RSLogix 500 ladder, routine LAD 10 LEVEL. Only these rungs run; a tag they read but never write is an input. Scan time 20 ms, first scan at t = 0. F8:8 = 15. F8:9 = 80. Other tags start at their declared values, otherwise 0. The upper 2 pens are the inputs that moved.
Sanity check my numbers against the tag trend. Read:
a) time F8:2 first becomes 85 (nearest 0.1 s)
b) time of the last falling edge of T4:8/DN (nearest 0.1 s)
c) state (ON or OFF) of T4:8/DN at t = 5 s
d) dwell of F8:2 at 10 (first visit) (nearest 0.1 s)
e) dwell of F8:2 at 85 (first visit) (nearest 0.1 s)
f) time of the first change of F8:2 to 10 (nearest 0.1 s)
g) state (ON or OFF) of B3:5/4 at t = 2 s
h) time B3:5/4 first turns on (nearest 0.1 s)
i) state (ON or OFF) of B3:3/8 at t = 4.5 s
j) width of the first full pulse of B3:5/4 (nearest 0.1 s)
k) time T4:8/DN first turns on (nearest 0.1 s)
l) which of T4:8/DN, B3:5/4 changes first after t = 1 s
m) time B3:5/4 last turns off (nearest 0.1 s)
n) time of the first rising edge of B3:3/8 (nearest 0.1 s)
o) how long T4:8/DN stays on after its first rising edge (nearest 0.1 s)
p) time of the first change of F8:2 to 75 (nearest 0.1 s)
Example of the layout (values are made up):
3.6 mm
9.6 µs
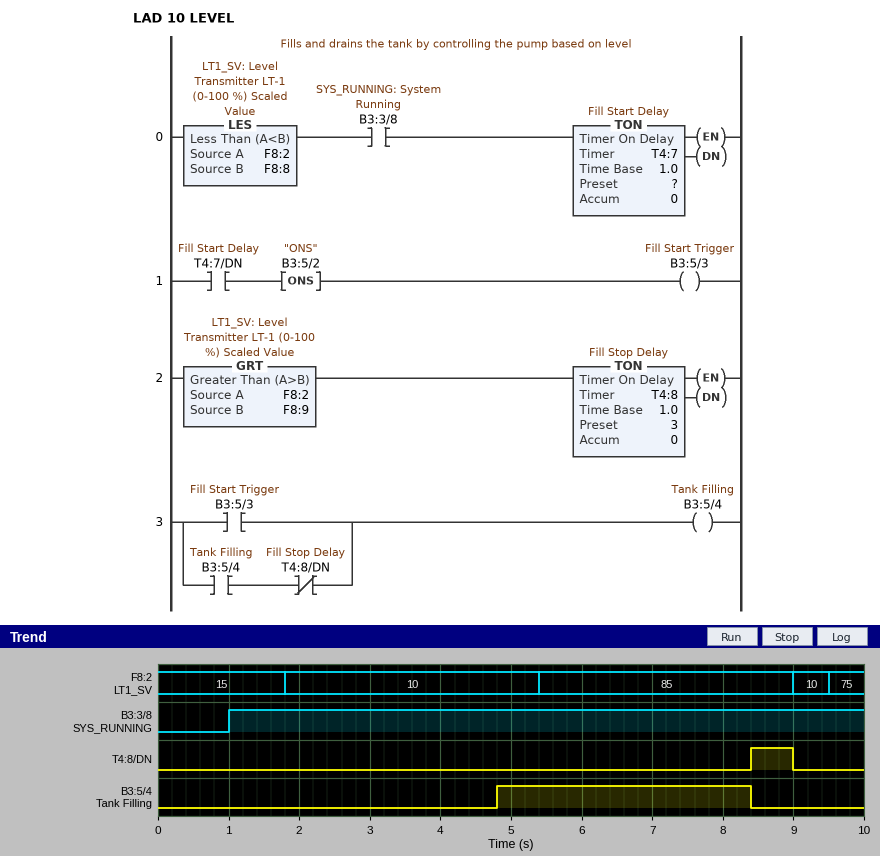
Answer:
5.4 s
9.0 s
OFF
3.6 s
3.6 s
1.8 s
OFF
4.8 s
ON
3.6 s
8.4 s
B3:5/4
8.4 s
1.0 s
0.6 s
9.5 s
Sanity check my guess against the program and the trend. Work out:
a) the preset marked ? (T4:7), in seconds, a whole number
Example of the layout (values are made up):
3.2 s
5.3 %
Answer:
3 s
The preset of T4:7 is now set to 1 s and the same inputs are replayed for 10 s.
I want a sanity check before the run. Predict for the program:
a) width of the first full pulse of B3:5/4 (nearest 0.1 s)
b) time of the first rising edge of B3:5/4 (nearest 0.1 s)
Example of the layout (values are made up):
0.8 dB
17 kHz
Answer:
5.6 s
2.8 s
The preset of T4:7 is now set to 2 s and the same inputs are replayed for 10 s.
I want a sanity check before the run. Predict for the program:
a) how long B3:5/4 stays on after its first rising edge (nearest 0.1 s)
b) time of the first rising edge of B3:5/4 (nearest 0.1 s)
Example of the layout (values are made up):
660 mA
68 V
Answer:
4.6 s
3.8 s
